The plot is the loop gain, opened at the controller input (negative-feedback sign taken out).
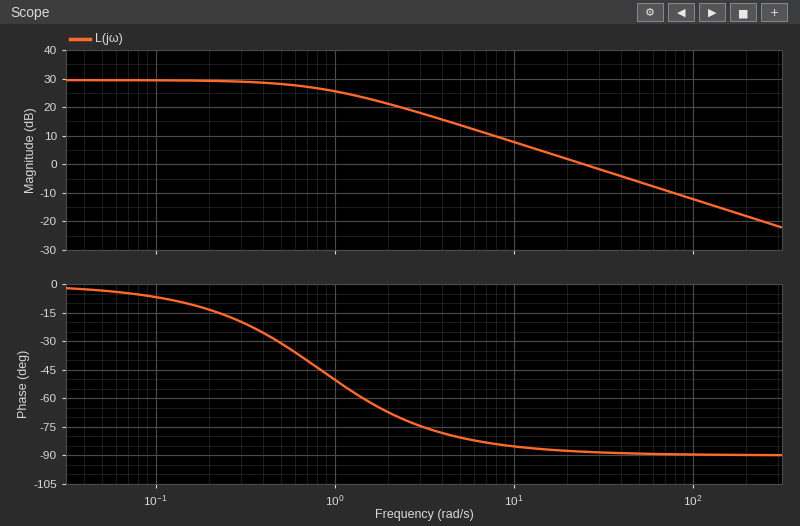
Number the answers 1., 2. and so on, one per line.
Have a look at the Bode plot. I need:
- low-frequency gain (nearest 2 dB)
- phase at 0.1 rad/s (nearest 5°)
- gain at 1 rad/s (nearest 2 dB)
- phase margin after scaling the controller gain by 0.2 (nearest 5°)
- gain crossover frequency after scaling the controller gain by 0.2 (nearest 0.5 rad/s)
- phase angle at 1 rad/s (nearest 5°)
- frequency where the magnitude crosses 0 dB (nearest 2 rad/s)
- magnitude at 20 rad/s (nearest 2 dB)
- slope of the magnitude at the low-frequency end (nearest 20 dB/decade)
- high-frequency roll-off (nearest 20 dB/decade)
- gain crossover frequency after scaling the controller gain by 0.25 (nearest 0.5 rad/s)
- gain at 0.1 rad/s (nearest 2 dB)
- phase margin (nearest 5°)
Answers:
1. 30 dB
2. -5°
3. 26 dB
4. 100°
5. 5.0 rad/s
6. -50°
7. 24 rad/s
8. 2 dB
9. 0 dB/decade
10. -20 dB/decade
11. 6.0 rad/s
12. 30 dB
13. 90°
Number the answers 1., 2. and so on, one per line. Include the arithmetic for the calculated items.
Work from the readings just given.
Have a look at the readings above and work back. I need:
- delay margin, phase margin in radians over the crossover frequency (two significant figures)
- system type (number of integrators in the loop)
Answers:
1. 90 × π / 180 / 24 = 0.065 s
2. 0
